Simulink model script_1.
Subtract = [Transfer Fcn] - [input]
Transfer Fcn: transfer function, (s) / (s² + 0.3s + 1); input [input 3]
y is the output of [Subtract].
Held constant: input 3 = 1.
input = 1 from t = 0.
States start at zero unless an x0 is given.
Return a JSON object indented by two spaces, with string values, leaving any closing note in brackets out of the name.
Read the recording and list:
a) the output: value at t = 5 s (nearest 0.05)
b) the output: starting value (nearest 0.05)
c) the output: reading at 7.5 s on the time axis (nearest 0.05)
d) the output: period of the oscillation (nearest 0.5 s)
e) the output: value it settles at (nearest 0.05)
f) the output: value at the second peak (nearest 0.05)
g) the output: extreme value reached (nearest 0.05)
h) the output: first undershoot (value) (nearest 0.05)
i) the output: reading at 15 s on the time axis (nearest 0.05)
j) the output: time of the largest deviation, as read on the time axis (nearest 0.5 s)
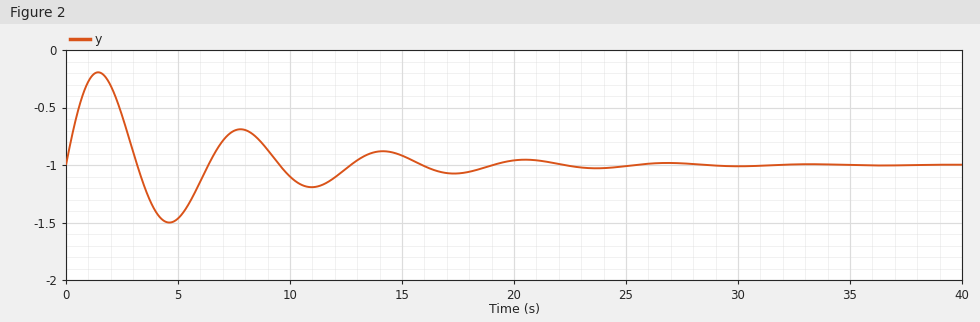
{
  "the output: value at t = 5 s": "-1.45",
  "the output: starting value": "-1.00",
  "the output: reading at 7.5 s on the time axis": "-0.70",
  "the output: period of the oscillation": "6.5 s",
  "the output: value it settles at": "-1.00",
  "the output: value at the second peak": "-0.70",
  "the output: extreme value reached": "-0.20",
  "the output: first undershoot (value)": "-1.50",
  "the output: reading at 15 s on the time axis": "-0.90",
  "the output: time of the largest deviation, as read on the time axis": "1.5 s"
}
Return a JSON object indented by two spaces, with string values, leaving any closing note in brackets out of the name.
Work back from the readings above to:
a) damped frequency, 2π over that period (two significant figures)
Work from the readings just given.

{
  "damped frequency, 2π over that period": "0.97 rad/s"
}
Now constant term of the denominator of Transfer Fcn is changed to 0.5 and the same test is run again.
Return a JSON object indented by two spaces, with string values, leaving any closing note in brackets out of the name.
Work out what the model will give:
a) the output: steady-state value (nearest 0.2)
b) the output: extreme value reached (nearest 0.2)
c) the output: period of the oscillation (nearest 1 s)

{
  "the output: steady-state value": "-1.0",
  "the output: extreme value reached": "0.0",
  "the output: period of the oscillation": "9 s"
}
